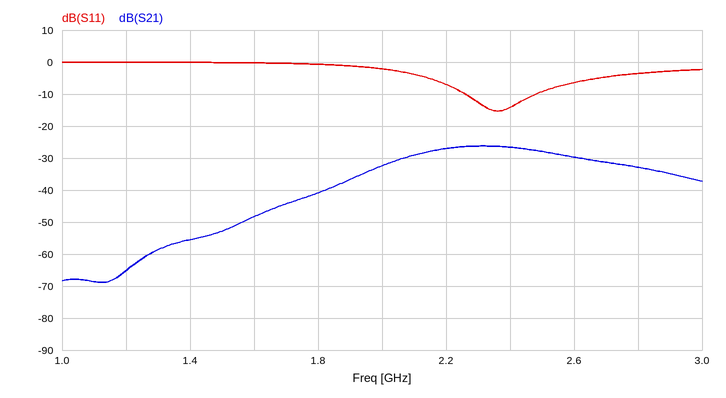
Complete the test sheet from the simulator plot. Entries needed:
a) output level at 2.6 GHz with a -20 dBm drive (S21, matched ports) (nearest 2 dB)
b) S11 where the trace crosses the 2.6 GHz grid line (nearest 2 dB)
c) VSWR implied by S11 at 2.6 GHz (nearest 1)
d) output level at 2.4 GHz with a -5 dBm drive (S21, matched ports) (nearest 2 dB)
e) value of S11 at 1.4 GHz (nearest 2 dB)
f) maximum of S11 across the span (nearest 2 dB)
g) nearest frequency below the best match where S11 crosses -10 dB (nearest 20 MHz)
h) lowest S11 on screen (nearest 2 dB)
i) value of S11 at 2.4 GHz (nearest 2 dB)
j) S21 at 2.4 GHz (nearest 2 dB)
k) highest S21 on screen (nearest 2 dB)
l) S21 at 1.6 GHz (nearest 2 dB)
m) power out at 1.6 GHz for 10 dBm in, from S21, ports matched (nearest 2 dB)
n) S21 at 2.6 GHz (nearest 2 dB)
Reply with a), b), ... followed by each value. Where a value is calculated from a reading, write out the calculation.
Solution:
a) -20 dBm + (-30 dB) = -50 dBm
b) -6 dB
c) |Γ| = 10^(-6/20) = 0.5012; VSWR = (1 + 0.5012)/(1 − 0.5012) ≈ 3
d) -5 dBm + (-26 dB) = -32 dBm
e) 0 dB
f) 0 dB
g) 2.26 GHz
h) -16 dB
i) -14 dB
j) -26 dB
k) -26 dB
l) -48 dB
m) 10 dBm + (-48 dB) = -38 dBm
n) -30 dB
